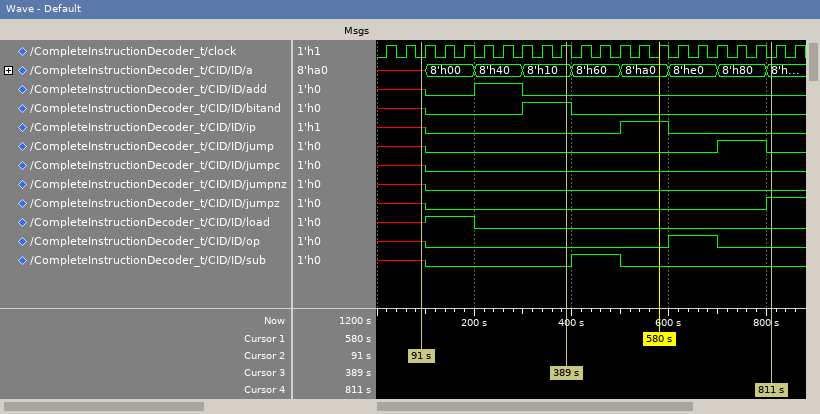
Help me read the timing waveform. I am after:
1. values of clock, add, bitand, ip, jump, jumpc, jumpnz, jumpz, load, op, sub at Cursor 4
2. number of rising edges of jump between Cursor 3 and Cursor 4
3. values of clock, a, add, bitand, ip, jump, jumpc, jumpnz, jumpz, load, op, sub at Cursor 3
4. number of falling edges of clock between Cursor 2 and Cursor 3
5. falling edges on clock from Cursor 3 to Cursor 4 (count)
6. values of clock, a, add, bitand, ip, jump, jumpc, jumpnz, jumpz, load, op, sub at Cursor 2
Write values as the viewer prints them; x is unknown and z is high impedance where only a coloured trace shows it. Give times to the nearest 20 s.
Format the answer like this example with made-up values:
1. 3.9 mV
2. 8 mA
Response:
1. clock=0, add=0, bitand=0, ip=0, jump=0, jumpc=0, jumpnz=0, jumpz=1, load=0, op=0, sub=0
2. 1
3. clock=1, a=8'h10, add=0, bitand=1, ip=0, jump=0, jumpc=0, jumpnz=0, jumpz=0, load=0, op=0, sub=0
4. 7
5. 11
6. clock=0, a=x, add=x, bitand=x, ip=x, jump=x, jumpc=x, jumpnz=x, jumpz=x, load=x, op=x, sub=x
